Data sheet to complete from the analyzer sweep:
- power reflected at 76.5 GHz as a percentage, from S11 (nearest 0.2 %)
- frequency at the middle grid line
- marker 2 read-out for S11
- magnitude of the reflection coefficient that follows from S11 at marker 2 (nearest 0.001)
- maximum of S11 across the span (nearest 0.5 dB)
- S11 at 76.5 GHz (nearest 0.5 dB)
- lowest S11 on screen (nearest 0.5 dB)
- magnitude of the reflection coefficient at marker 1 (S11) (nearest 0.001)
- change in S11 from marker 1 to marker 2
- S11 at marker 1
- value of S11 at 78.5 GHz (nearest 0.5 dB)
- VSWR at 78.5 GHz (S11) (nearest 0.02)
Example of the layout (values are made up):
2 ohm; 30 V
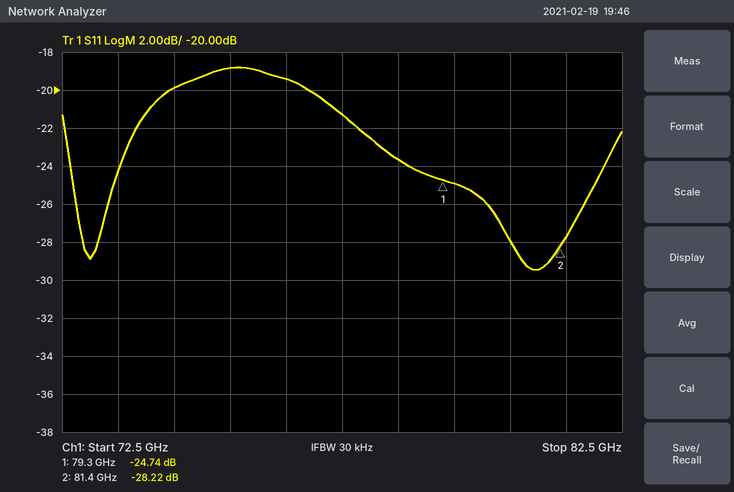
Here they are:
1.2 %; 77.5 GHz; -28.22 dB; 0.039; -19.0 dB; -19.5 dB; -29.5 dB; 0.058; -3.48 dB; -24.74 dB; -23.5 dB; 1.14
